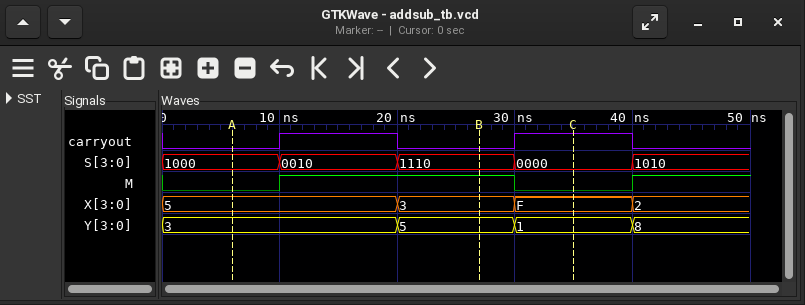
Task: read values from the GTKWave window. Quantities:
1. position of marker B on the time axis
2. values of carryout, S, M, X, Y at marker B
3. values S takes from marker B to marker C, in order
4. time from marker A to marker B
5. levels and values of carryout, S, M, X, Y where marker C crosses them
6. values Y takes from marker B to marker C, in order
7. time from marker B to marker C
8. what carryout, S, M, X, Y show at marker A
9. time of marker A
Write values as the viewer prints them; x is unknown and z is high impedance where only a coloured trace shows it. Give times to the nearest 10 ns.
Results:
30 ns
carryout=0, S=1110, M=1, X=3, Y=5
1110, 0000
20 ns
carryout=1, S=0000, M=0, X=F, Y=1
5, 1
10 ns
carryout=0, S=1000, M=0, X=5, Y=3
10 ns
